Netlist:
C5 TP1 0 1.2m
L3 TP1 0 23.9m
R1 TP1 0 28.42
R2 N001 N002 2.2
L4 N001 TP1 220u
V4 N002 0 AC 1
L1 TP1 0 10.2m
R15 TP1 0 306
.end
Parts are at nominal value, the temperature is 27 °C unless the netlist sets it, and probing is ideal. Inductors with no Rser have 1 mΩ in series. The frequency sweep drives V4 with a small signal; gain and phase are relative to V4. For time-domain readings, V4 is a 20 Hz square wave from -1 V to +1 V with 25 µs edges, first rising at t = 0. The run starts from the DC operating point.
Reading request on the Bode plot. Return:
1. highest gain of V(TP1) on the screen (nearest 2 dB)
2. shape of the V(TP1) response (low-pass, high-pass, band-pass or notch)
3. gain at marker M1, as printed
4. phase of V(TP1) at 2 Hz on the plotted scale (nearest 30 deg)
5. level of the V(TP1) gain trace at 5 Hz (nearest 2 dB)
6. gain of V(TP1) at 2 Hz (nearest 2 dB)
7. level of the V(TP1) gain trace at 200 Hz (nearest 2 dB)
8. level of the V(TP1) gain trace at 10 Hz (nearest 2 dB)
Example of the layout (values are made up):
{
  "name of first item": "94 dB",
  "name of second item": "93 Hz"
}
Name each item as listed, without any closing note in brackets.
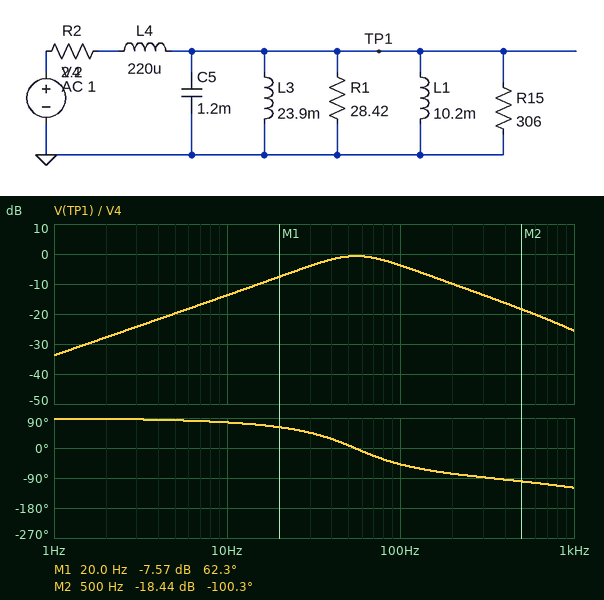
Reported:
{
  "highest gain of V(TP1) on the screen": "0 dB",
  "shape of the V(TP1) response": "band-pass",
  "gain at marker M1, as printed": "-7.57 dB",
  "phase of V(TP1) at 2 Hz on the plotted scale": "90 deg",
  "level of the V(TP1) gain trace at 5 Hz": "-20 dB",
  "gain of V(TP1) at 2 Hz": "-28 dB",
  "level of the V(TP1) gain trace at 200 Hz": "-10 dB",
  "level of the V(TP1) gain trace at 10 Hz": "-14 dB"
}
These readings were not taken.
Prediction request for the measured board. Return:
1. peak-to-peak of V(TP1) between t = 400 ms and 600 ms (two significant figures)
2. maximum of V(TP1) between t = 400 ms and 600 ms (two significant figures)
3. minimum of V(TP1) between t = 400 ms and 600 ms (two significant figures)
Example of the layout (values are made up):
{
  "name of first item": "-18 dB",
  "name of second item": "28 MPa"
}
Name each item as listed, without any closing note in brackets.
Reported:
{
  "peak-to-peak of V(TP1) between t = 400 ms and 600 ms": "2.2 V",
  "maximum of V(TP1) between t = 400 ms and 600 ms": "1.1 V",
  "minimum of V(TP1) between t = 400 ms and 600 ms": "-1.1 V"
}
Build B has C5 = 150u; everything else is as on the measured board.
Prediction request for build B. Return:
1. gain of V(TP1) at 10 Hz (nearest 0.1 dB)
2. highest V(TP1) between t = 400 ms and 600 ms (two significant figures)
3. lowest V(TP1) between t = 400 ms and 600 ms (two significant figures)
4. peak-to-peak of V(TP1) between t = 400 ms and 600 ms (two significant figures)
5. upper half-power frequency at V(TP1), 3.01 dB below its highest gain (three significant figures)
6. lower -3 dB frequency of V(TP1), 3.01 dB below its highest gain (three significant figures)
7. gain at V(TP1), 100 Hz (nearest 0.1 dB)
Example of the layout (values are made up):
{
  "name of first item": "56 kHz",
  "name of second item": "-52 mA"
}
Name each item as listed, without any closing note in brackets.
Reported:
{
  "gain of V(TP1) at 10 Hz": "-14.0 dB",
  "highest V(TP1) between t = 400 ms and 600 ms": "1.7 V",
  "lowest V(TP1) between t = 400 ms and 600 ms": "-1.7 V",
  "peak-to-peak of V(TP1) between t = 400 ms and 600 ms": "3.3 V",
  "upper half-power frequency at V(TP1), 3.01 dB below its highest gain": "718 Hz",
  "lower -3 dB frequency of V(TP1), 3.01 dB below its highest gain": "43.2 Hz",
  "gain at V(TP1), 100 Hz": "-1.1 dB"
}
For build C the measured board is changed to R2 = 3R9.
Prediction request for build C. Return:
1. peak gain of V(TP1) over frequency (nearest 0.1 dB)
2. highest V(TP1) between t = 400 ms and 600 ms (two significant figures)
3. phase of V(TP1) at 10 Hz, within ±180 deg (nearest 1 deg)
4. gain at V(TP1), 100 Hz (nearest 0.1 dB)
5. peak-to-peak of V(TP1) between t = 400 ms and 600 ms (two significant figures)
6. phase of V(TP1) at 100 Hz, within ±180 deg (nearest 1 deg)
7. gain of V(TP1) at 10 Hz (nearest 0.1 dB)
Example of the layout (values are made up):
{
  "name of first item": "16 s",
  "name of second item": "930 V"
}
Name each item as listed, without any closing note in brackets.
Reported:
{
  "peak gain of V(TP1) over frequency": "-1.2 dB",
  "highest V(TP1) between t = 400 ms and 600 ms": "780 mV",
  "phase of V(TP1) at 10 Hz, within ±180 deg": "82 deg",
  "gain at V(TP1), 100 Hz": "-7.4 dB",
  "peak-to-peak of V(TP1) between t = 400 ms and 600 ms": "1.6 V",
  "phase of V(TP1) at 100 Hz, within ±180 deg": "-63 deg",
  "gain of V(TP1) at 10 Hz": "-18.6 dB"
}
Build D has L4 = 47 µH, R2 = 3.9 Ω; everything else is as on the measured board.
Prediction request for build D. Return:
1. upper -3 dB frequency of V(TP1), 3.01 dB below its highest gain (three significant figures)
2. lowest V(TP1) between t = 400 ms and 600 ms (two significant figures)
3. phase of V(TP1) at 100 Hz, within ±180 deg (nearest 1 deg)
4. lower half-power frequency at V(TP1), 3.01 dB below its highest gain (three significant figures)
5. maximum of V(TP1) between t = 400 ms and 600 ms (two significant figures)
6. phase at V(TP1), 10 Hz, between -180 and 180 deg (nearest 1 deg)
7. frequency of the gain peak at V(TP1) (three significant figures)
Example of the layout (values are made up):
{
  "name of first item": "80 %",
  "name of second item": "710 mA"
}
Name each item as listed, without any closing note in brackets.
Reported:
{
  "upper -3 dB frequency of V(TP1), 3.01 dB below its highest gain": "77.4 Hz",
  "lowest V(TP1) between t = 400 ms and 600 ms": "-780 mV",
  "phase of V(TP1) at 100 Hz, within ±180 deg": "-61 deg",
  "lower half-power frequency at V(TP1), 3.01 dB below its highest gain": "38.2 Hz",
  "maximum of V(TP1) between t = 400 ms and 600 ms": "780 mV",
  "phase at V(TP1), 10 Hz, between -180 and 180 deg": "82 deg",
  "frequency of the gain peak at V(TP1)": "54.4 Hz"
}
